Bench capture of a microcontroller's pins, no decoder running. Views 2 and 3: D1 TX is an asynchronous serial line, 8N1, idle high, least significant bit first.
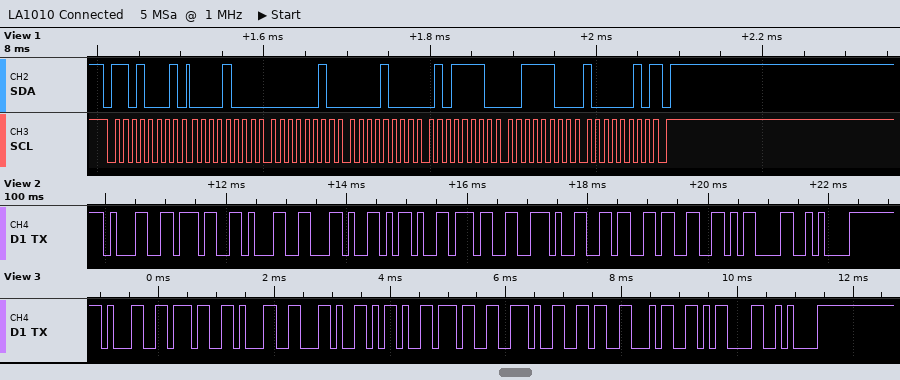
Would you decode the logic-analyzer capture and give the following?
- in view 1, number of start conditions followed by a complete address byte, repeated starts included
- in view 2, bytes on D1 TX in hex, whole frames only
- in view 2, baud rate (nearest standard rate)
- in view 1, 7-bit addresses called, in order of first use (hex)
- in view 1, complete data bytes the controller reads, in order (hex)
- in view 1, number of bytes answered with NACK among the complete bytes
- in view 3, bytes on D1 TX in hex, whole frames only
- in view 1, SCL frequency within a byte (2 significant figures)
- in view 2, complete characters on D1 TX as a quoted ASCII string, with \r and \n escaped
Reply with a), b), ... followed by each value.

a) 1
b) 31 37 31 2C 2D 37 2E 36 33 0D 0A
c) 9600 baud
d) 0x68
e) 08 02 08 5E 3C 82
f) 1
g) 31 37 31 2C 2D 37 2E 36 34 0D 0A
h) 100 kHz
i) "171,-7.63\r\n"
